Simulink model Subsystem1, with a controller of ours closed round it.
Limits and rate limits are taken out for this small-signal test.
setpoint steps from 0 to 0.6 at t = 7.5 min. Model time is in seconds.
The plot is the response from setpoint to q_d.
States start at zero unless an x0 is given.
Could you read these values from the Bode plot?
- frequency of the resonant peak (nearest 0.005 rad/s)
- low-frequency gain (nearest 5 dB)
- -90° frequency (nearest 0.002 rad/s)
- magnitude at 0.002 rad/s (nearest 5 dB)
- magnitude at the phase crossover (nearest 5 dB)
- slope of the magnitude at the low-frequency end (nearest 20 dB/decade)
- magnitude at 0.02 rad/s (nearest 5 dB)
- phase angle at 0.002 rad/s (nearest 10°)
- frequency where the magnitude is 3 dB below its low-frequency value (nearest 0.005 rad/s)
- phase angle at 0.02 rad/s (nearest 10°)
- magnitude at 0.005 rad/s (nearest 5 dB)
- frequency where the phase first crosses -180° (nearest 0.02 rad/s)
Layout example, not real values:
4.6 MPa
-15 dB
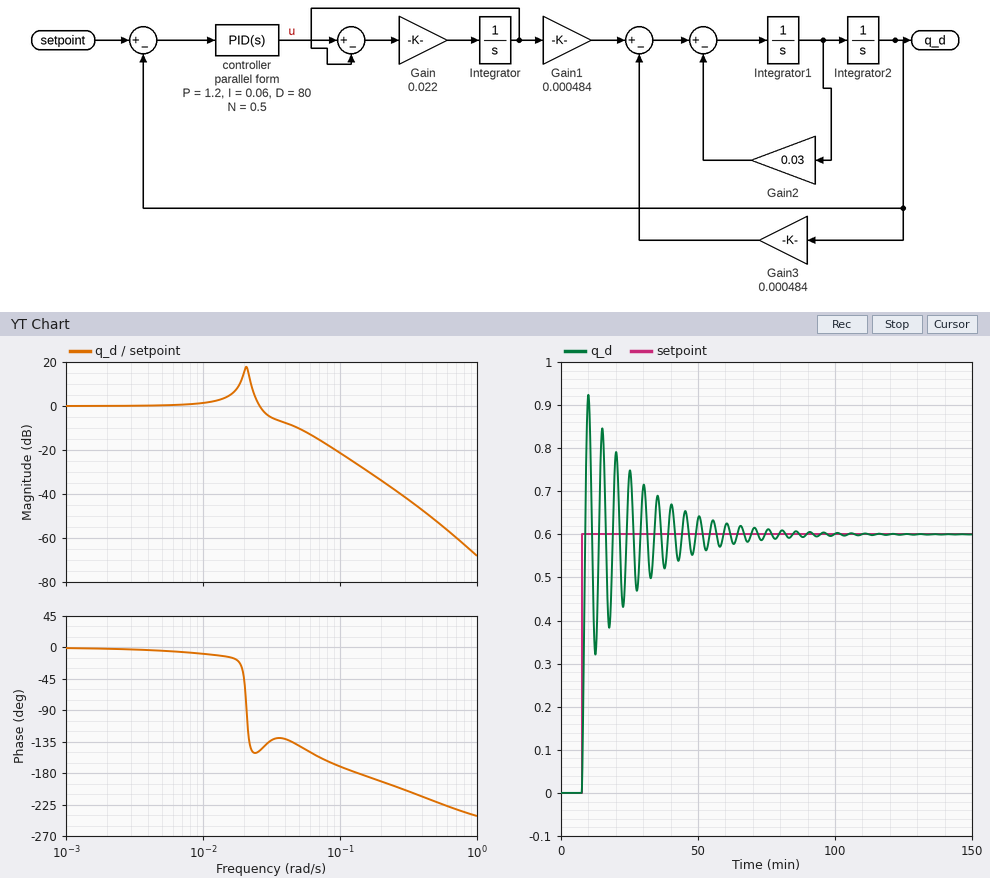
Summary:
0.020 rad/s
0 dB
0.020 rad/s
0 dB
-25 dB
0 dB/decade
15 dB
0°
0.030 rad/s
-50°
0 dB
0.14 rad/s
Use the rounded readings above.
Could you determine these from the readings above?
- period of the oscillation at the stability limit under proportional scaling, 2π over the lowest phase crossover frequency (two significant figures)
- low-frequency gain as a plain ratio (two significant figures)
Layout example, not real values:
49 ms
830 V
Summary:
45 s
1.0
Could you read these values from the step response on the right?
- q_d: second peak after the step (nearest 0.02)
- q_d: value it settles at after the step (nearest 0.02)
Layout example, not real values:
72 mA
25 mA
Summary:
0.84
0.60
